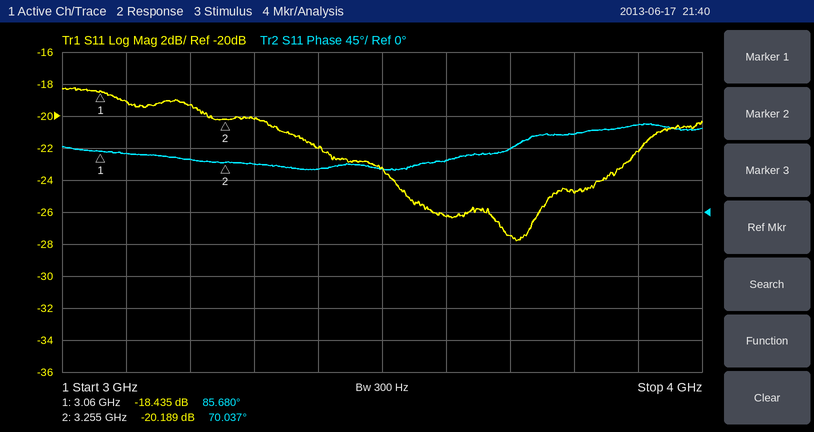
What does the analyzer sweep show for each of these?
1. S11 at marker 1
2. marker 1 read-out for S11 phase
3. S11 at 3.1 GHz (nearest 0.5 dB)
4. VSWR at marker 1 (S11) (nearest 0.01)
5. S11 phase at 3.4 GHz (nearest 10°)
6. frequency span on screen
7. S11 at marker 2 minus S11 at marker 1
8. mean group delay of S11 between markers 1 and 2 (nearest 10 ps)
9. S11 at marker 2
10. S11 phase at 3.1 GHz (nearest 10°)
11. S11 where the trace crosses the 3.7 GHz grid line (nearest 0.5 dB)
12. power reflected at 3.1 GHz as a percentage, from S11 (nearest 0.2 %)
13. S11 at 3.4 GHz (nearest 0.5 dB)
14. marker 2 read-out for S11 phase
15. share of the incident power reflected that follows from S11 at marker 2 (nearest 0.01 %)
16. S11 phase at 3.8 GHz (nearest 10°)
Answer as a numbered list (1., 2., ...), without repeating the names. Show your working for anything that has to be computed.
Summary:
1. -18.435 dB
2. 85.680°
3. -19.0 dB
4. (1 + 0.1197)/(1 − 0.1197) ≈ 1.27
5. 60°
6. 1 GHz
7. -20.189 − (-18.435) = -1.754 dB
8. −(70.037° − (85.68°))/(360° × 195 MHz) ≈ 223 ps, so 220 ps to the nearest 10 ps
9. -20.189 dB
10. 80°
11. -27.5 dB
12. 10^(-19/10) ≈ 1.26 %, so 1.2 % to the nearest 0.2 %
13. -22.0 dB
14. 70.037°
15. 10^(-20.189/10) ≈ 0.96 %
16. 110°
